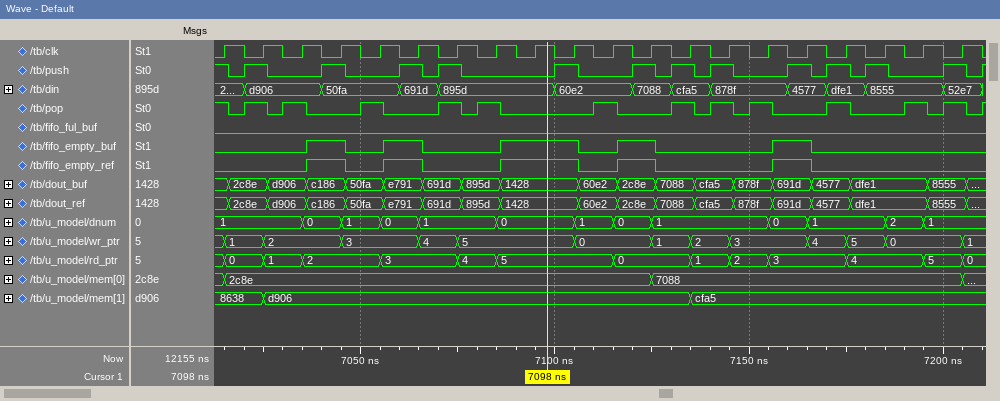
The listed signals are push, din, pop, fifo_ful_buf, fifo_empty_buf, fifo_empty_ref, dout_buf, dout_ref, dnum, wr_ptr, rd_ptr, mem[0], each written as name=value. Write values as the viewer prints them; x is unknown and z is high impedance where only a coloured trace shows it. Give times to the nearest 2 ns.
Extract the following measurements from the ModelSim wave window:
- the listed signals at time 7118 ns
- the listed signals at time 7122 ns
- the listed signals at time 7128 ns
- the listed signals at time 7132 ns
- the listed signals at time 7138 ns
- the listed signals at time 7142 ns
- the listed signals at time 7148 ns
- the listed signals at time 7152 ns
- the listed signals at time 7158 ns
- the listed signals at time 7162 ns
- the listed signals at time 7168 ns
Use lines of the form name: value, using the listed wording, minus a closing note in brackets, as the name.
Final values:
the listed signals at time 7118 ns: push=0, din=60e2, pop=0, fifo_ful_buf=0, fifo_empty_buf=1, fifo_empty_ref=1, dout_buf=2c8e, dout_ref=2c8e, dnum=0, wr_ptr=0, rd_ptr=0, mem[0]=2c8e
the listed signals at time 7122 ns: push=1, din=7088, pop=0, fifo_ful_buf=0, fifo_empty_buf=1, fifo_empty_ref=1, dout_buf=2c8e, dout_ref=2c8e, dnum=0, wr_ptr=0, rd_ptr=0, mem[0]=2c8e
the listed signals at time 7128 ns: push=0, din=7088, pop=0, fifo_ful_buf=0, fifo_empty_buf=0, fifo_empty_ref=0, dout_buf=7088, dout_ref=7088, dnum=1, wr_ptr=1, rd_ptr=0, mem[0]=7088
the listed signals at time 7132 ns: push=1, din=cfa5, pop=1, fifo_ful_buf=0, fifo_empty_buf=0, fifo_empty_ref=0, dout_buf=7088, dout_ref=7088, dnum=1, wr_ptr=1, rd_ptr=0, mem[0]=7088
the listed signals at time 7138 ns: push=0, din=cfa5, pop=0, fifo_ful_buf=0, fifo_empty_buf=0, fifo_empty_ref=0, dout_buf=cfa5, dout_ref=cfa5, dnum=1, wr_ptr=2, rd_ptr=1, mem[0]=7088
the listed signals at time 7142 ns: push=1, din=878f, pop=1, fifo_ful_buf=0, fifo_empty_buf=0, fifo_empty_ref=0, dout_buf=cfa5, dout_ref=cfa5, dnum=1, wr_ptr=2, rd_ptr=1, mem[0]=7088
the listed signals at time 7148 ns: push=0, din=878f, pop=0, fifo_ful_buf=0, fifo_empty_buf=0, fifo_empty_ref=0, dout_buf=878f, dout_ref=878f, dnum=1, wr_ptr=3, rd_ptr=2, mem[0]=7088
the listed signals at time 7152 ns: push=0, din=878f, pop=1, fifo_ful_buf=0, fifo_empty_buf=0, fifo_empty_ref=0, dout_buf=878f, dout_ref=878f, dnum=1, wr_ptr=3, rd_ptr=2, mem[0]=7088
the listed signals at time 7158 ns: push=0, din=878f, pop=0, fifo_ful_buf=0, fifo_empty_buf=1, fifo_empty_ref=1, dout_buf=691d, dout_ref=691d, dnum=0, wr_ptr=3, rd_ptr=3, mem[0]=7088
the listed signals at time 7162 ns: push=1, din=4577, pop=0, fifo_ful_buf=0, fifo_empty_buf=1, fifo_empty_ref=1, dout_buf=691d, dout_ref=691d, dnum=0, wr_ptr=3, rd_ptr=3, mem[0]=7088
the listed signals at time 7168 ns: push=0, din=4577, pop=0, fifo_ful_buf=0, fifo_empty_buf=0, fifo_empty_ref=0, dout_buf=4577, dout_ref=4577, dnum=1, wr_ptr=4, rd_ptr=3, mem[0]=7088
